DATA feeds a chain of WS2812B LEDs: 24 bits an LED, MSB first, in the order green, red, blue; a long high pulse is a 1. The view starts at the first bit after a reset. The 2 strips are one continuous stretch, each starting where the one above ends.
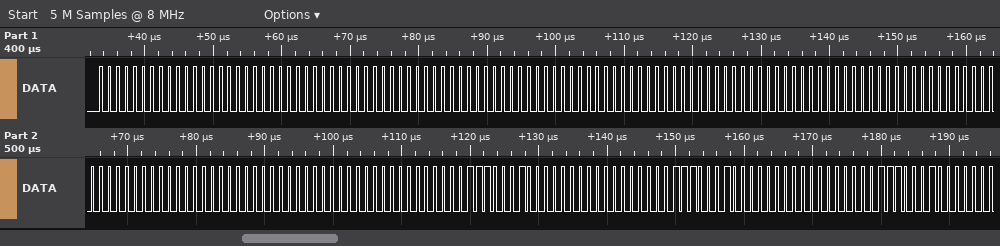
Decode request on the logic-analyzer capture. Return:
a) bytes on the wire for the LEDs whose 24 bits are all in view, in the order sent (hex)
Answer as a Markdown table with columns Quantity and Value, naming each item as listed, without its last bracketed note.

| Quantity | Value |
|---|---|
| bytes on the wire for the LEDs whose 24 bits are all in view, in the order sent | 00 00 00 00 00 00 00 00 00 00 00 00 00 00 00 00 00 00 07 10 00 07 10 00 |
